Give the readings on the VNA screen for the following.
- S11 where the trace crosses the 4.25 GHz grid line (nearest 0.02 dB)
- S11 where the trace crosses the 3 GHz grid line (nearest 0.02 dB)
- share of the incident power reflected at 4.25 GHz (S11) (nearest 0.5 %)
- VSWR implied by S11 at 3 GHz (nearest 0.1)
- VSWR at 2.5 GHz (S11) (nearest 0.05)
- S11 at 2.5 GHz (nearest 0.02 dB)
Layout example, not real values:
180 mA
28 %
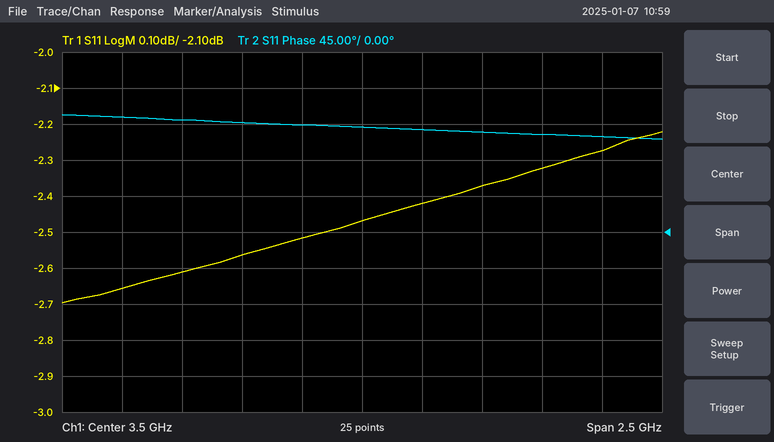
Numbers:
-2.32 dB
-2.56 dB
58.5 %
6.8
6.60
-2.66 dB
